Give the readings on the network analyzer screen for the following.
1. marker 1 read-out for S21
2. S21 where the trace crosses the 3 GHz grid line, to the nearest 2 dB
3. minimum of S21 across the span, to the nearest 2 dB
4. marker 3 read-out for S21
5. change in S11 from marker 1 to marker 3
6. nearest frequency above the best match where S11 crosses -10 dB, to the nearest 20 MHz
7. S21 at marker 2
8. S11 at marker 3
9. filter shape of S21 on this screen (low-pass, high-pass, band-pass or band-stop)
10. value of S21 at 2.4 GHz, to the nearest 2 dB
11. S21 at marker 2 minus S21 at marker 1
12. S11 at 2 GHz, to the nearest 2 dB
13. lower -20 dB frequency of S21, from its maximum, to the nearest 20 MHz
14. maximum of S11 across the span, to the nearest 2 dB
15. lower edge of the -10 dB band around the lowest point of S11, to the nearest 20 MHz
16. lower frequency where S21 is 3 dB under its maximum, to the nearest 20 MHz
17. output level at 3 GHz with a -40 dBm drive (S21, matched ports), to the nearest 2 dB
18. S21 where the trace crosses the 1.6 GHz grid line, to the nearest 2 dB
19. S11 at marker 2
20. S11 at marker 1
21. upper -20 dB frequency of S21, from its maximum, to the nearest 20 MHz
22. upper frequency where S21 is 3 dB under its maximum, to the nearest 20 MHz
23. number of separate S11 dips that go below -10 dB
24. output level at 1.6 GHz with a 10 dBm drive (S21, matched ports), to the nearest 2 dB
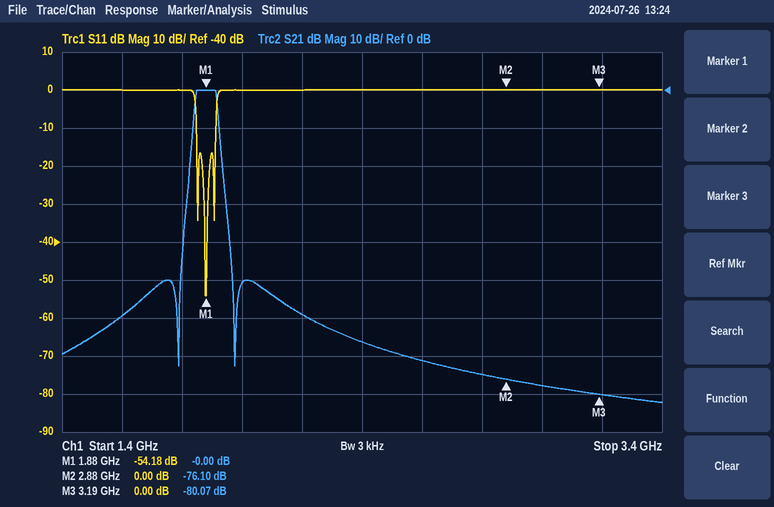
-0.00 dB
-78 dB
-82 dB
-80.07 dB
54.18 dB
1.92 GHz
-76.10 dB
0.00 dB
band-pass
-66 dB
-76.10 dB
0 dB
1.82 GHz
0 dB
1.84 GHz
1.84 GHz
-118 dBm
-60 dB
0.00 dB
-54.18 dB
1.94 GHz
1.92 GHz
3
-50 dBm
